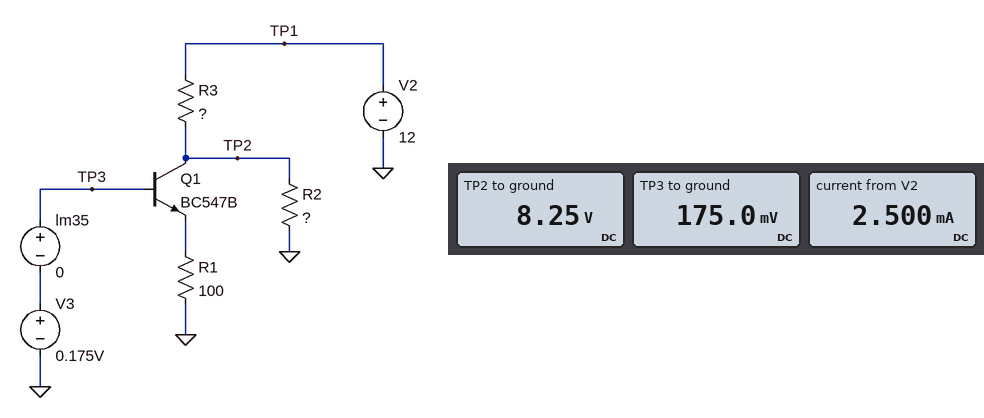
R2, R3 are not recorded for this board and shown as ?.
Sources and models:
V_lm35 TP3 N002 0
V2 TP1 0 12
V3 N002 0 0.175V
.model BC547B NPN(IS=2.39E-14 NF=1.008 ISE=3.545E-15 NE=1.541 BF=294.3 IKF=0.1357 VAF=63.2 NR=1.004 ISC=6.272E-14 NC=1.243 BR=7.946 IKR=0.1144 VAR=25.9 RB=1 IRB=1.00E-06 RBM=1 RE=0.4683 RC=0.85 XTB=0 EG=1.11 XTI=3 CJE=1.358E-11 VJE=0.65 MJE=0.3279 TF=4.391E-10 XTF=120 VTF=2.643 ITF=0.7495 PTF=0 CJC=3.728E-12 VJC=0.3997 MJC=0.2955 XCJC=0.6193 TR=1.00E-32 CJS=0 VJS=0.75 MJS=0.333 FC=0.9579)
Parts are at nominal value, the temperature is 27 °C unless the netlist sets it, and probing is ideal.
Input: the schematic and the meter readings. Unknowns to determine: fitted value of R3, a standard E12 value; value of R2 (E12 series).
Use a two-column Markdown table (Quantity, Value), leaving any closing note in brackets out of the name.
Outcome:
| Quantity | Value |
|---|---|
| fitted value of R3, a standard E12 value | 1.5 kΩ |
| value of R2 | 3.3 kΩ |
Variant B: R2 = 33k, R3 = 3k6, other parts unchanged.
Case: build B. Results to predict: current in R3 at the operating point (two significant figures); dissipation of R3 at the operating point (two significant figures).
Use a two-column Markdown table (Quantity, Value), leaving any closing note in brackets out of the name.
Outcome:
| Quantity | Value |
|---|---|
| current in R3 at the operating point | 330 µA |
| dissipation of R3 at the operating point | 390 µW |
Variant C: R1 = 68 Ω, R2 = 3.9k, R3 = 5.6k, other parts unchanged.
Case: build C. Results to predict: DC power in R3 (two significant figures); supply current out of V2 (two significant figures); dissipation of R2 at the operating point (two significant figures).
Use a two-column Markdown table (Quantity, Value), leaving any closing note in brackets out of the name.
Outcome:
| Quantity | Value |
|---|---|
| DC power in R3 | 8.9 mW |
| supply current out of V2 | 1.3 mA |
| dissipation of R2 at the operating point | 6.2 mW |
